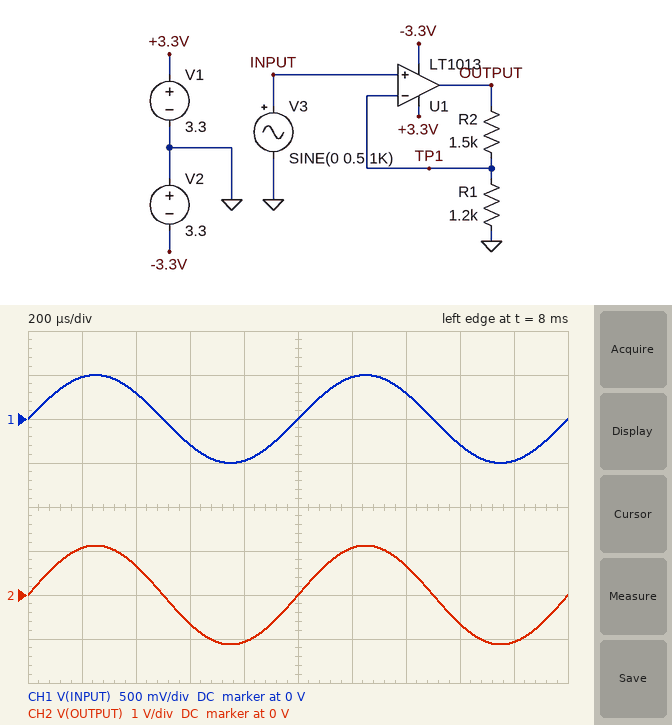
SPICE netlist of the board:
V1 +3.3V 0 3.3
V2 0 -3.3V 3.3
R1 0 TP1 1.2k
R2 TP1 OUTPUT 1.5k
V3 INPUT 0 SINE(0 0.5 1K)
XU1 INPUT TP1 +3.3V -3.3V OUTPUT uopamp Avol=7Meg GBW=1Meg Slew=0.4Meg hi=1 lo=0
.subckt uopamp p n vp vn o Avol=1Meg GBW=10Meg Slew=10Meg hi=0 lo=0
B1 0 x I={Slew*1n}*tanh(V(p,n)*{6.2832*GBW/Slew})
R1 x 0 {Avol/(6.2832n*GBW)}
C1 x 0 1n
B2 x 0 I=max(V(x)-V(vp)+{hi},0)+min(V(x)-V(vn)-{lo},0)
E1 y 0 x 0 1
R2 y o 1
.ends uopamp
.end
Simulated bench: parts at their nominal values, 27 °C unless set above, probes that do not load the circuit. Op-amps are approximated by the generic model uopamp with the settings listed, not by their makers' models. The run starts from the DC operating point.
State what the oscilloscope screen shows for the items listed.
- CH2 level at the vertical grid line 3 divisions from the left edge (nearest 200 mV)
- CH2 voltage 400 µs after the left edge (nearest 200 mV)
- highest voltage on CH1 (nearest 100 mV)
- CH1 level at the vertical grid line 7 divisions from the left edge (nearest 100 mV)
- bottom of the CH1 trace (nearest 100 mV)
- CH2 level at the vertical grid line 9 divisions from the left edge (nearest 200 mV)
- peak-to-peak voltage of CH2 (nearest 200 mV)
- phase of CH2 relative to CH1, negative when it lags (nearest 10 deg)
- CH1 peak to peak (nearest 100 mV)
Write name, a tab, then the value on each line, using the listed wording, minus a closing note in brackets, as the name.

CH2 level at the vertical grid line 3 divisions from the left edge	-600 mV
CH2 voltage 400 µs after the left edge	600 mV
highest voltage on CH1	500 mV
CH1 level at the vertical grid line 7 divisions from the left edge	300 mV
bottom of the CH1 trace	-500 mV
CH2 level at the vertical grid line 9 divisions from the left edge	-1.0 V
peak-to-peak voltage of CH2	2.2 V
phase of CH2 relative to CH1, negative when it lags	0 deg
CH1 peak to peak	1.0 V
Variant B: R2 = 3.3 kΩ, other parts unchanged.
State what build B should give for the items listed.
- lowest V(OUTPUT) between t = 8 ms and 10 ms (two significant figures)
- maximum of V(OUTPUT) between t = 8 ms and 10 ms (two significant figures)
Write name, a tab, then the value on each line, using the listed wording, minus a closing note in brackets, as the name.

lowest V(OUTPUT) between t = 8 ms and 10 ms	-1.9 V
maximum of V(OUTPUT) between t = 8 ms and 10 ms	1.9 V
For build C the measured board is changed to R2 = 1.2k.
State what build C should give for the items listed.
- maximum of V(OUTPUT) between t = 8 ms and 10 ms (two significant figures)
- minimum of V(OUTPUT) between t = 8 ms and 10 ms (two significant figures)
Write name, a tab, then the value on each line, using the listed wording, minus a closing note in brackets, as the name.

maximum of V(OUTPUT) between t = 8 ms and 10 ms	1.0 V
minimum of V(OUTPUT) between t = 8 ms and 10 ms	-1.0 V
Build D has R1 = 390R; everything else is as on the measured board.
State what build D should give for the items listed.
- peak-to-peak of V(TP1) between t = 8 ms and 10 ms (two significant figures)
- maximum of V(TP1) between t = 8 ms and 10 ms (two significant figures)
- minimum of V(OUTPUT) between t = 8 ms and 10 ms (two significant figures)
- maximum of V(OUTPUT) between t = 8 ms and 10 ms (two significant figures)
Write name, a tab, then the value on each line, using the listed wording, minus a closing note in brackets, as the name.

peak-to-peak of V(TP1) between t = 8 ms and 10 ms	970 mV
maximum of V(TP1) between t = 8 ms and 10 ms	470 mV
minimum of V(OUTPUT) between t = 8 ms and 10 ms	-2.4 V
maximum of V(OUTPUT) between t = 8 ms and 10 ms	2.3 V
